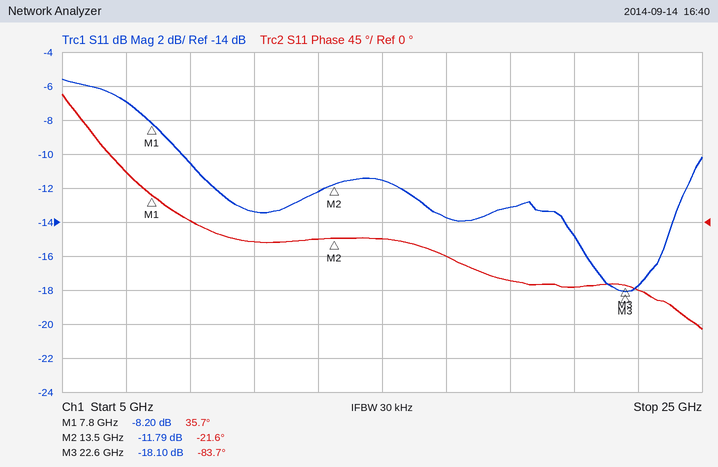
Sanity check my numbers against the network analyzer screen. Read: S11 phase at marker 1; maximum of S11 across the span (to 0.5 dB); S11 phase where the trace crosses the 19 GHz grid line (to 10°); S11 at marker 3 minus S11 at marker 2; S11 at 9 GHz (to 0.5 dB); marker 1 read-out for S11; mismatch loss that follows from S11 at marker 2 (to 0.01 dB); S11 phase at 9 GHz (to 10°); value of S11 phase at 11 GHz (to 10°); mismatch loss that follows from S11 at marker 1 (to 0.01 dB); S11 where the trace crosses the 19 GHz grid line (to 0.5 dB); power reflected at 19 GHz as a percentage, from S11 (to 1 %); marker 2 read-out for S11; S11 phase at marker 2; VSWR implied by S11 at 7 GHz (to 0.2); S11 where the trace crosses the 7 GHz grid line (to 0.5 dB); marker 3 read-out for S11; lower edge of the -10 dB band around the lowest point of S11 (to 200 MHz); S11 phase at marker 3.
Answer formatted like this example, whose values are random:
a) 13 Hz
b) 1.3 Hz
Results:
a) 35.7°
b) -5.5 dB
c) -80°
d) -6.31 dB
e) -10.5 dB
f) -8.20 dB
g) 0.30 dB
h) 0°
i) -30°
j) 0.71 dB
k) -13.0 dB
l) 5 %
m) -11.79 dB
n) -21.6°
o) 2.6
p) -7.0 dB
q) -18.10 dB
r) 8.8 GHz
s) -83.7°
